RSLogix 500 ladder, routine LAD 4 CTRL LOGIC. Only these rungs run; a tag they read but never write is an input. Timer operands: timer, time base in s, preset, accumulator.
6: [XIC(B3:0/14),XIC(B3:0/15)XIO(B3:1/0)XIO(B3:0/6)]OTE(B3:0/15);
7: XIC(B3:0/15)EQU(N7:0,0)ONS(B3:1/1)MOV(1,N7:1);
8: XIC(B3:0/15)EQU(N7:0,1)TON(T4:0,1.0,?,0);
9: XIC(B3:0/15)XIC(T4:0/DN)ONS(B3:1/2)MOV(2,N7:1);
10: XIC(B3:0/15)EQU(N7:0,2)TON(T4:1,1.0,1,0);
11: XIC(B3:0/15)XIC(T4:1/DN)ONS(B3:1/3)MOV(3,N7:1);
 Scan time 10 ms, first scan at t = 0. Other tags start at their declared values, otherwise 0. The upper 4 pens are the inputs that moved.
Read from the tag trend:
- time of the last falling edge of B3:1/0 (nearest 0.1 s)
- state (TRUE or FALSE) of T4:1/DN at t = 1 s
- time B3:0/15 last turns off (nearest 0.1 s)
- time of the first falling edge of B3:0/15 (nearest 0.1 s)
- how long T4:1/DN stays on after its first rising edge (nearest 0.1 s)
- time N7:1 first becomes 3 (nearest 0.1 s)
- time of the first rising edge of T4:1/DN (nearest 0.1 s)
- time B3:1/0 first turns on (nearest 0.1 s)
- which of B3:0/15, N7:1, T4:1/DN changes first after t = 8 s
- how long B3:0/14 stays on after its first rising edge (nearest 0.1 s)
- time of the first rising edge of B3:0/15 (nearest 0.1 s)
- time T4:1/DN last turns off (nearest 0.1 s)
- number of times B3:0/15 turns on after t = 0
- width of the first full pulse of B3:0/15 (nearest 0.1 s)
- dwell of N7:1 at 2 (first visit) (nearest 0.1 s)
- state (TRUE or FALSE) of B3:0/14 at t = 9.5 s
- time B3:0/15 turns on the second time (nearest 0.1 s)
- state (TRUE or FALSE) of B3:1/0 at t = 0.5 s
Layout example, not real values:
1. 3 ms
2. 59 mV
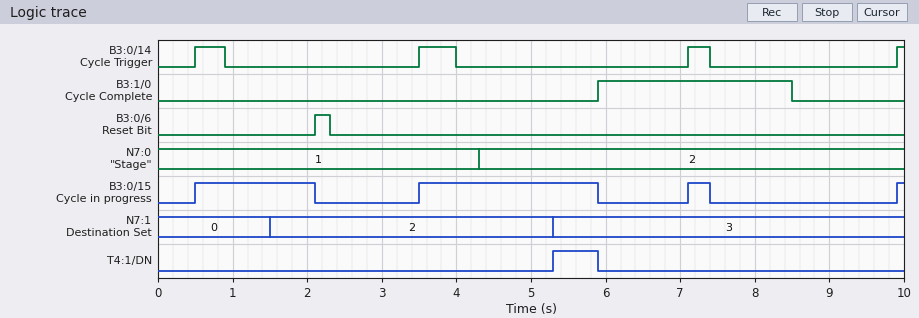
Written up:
1. 8.5 s
2. FALSE
3. 7.4 s
4. 2.1 s
5. 0.6 s
6. 5.3 s
7. 5.3 s
8. 5.9 s
9. B3:0/15
10. 0.4 s
11. 0.5 s
12. 5.9 s
13. 4
14. 1.6 s
15. 3.8 s
16. FALSE
17. 3.5 s
18. FALSE
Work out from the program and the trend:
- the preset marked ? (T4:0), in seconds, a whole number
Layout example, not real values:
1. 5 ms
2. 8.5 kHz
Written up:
1. 1 s
